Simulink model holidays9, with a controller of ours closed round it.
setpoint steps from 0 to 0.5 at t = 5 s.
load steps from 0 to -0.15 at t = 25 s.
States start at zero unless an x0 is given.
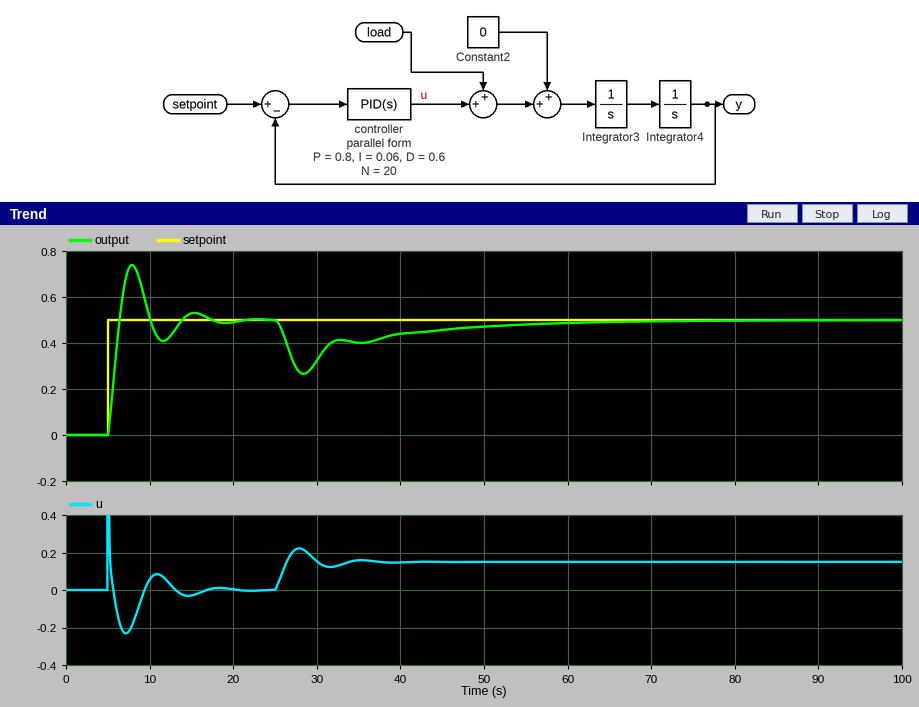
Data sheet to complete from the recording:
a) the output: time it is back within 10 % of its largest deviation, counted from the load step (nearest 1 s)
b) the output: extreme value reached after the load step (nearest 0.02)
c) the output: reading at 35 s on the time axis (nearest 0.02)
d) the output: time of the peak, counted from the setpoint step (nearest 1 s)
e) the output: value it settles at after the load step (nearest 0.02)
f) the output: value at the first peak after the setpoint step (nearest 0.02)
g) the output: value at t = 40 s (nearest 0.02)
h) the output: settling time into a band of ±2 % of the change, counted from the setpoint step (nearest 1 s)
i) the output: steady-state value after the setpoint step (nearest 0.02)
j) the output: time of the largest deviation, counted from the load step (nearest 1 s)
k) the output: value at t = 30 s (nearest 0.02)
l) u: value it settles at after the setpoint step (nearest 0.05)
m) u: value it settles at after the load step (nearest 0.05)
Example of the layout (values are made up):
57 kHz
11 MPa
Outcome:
28 s
0.26
0.40
3 s
0.50
0.74
0.44
15 s
0.50
3 s
0.32
0.00
0.15
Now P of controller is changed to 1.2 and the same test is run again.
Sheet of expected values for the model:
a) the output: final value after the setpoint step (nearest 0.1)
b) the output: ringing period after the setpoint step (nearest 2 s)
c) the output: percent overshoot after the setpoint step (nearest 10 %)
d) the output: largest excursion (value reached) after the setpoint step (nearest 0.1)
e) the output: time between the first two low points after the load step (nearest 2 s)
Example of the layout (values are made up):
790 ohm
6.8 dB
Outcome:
0.5
6 s
50 %
0.8
6 s
